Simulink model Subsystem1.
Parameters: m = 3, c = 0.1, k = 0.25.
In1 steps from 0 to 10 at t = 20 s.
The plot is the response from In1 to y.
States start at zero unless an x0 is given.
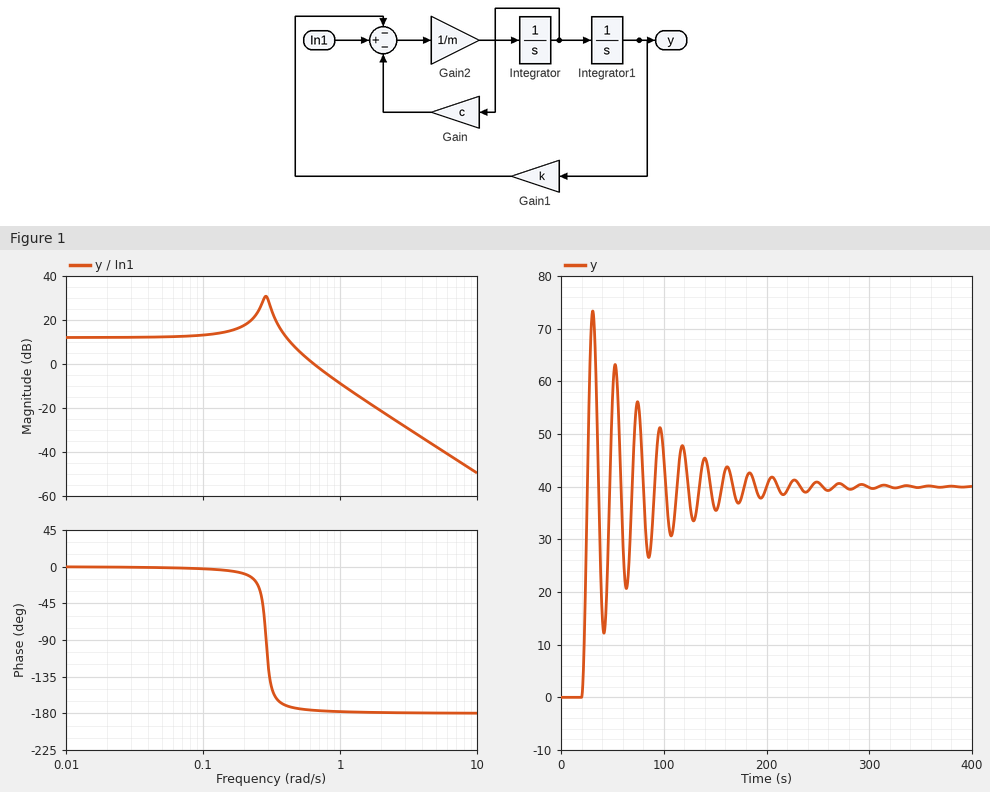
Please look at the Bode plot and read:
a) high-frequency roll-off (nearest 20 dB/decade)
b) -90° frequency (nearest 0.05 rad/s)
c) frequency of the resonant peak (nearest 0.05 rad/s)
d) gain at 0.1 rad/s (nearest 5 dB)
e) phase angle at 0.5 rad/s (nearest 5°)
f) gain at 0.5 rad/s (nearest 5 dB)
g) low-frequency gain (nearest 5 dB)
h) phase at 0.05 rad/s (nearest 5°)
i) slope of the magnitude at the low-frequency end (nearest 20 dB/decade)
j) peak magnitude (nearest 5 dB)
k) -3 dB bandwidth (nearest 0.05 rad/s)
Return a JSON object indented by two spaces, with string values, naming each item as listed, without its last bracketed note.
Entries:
{
  "high-frequency roll-off": "-40 dB/decade",
  "-90° frequency": "0.30 rad/s",
  "frequency of the resonant peak": "0.30 rad/s",
  "gain at 0.1 rad/s": "15 dB",
  "phase angle at 0.5 rad/s": "-175°",
  "gain at 0.5 rad/s": "5 dB",
  "low-frequency gain": "10 dB",
  "phase at 0.05 rad/s": "0°",
  "slope of the magnitude at the low-frequency end": "0 dB/decade",
  "peak magnitude": "30 dB",
  "-3 dB bandwidth": "0.45 rad/s"
}
